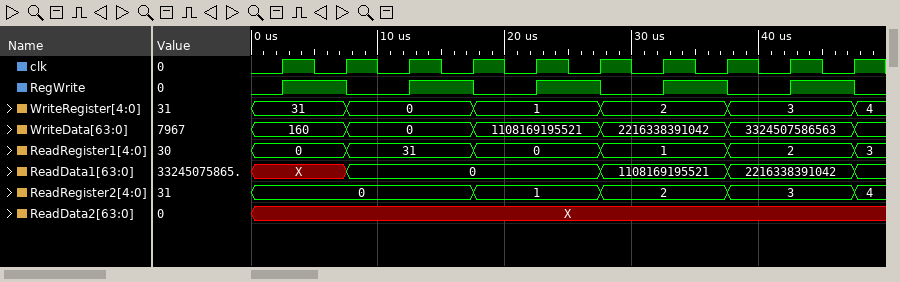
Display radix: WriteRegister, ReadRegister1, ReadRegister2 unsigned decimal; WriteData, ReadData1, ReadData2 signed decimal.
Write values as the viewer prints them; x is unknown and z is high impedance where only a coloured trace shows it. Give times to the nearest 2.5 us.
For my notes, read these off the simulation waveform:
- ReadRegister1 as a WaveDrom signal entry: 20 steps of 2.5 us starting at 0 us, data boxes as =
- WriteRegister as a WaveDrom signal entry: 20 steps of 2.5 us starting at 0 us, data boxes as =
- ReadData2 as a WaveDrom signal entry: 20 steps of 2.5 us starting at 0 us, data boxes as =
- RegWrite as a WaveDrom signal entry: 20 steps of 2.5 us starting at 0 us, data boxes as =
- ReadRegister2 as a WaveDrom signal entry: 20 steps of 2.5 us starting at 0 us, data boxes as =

{name: 'ReadRegister1', wave: '=..=...=...=...=...=', data: '0 31 0 1 2 3'}
{name: 'WriteRegister', wave: '=..=...=...=...=...=', data: '31 0 1 2 3 4'}
{name: 'ReadData2', wave: 'x...................'}
{name: 'RegWrite', wave: '01.0.1.0.1.0.1.0.1.0'}
{name: 'ReadRegister2', wave: '=......=...=...=...=', data: '0 1 2 3 4'}
